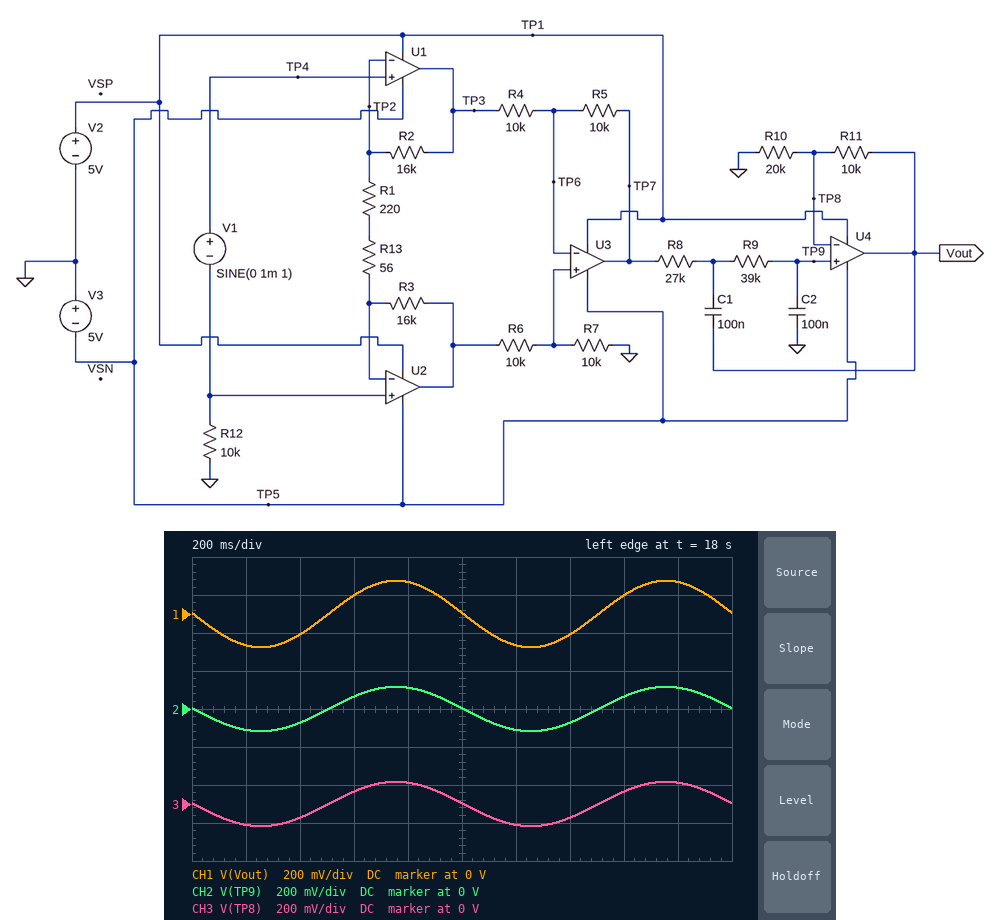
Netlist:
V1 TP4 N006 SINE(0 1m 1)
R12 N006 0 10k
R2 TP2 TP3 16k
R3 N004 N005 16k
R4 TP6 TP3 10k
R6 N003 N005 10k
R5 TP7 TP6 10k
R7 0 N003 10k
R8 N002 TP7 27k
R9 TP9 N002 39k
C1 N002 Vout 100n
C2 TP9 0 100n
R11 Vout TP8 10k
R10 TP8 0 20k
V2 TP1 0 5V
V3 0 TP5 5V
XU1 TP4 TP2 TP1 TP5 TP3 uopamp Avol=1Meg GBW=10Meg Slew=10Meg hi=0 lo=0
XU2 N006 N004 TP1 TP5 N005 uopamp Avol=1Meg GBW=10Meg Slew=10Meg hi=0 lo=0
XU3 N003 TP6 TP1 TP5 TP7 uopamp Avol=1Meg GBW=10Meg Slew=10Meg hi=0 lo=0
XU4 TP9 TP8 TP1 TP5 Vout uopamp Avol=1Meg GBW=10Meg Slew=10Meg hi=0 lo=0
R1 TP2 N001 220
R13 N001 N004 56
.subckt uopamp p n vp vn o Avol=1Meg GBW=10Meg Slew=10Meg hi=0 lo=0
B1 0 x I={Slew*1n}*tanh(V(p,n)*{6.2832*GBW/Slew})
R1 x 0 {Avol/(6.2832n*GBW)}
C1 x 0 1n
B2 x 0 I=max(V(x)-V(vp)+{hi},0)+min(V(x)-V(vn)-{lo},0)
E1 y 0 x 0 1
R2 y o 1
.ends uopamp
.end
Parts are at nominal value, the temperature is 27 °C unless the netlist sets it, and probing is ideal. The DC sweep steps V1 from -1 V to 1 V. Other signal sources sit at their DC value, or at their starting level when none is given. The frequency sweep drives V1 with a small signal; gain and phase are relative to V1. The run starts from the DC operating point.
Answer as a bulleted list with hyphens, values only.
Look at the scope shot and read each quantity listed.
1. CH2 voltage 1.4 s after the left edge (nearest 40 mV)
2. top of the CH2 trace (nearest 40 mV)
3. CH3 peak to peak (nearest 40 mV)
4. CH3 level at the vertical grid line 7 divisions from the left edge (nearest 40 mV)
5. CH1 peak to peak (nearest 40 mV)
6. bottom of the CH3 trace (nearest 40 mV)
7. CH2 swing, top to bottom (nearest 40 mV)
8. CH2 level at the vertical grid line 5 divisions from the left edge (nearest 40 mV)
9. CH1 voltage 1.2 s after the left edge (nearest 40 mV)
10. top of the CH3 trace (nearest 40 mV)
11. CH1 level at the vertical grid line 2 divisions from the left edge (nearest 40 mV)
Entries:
- -80 mV
- 120 mV
- 240 mV
- -80 mV
- 360 mV
- -120 mV
- 240 mV
- 0 V
- -160 mV
- 120 mV
- -120 mV
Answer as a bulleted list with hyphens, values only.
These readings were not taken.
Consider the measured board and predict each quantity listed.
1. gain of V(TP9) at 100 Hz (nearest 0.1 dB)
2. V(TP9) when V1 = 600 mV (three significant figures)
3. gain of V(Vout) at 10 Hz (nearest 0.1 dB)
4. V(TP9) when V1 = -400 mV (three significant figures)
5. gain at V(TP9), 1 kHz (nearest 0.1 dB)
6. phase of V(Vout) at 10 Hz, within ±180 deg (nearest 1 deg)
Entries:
- 28.2 dB
- -5.01 V
- 44.8 dB
- 5.01 V
- -11.0 dB
- 161 deg
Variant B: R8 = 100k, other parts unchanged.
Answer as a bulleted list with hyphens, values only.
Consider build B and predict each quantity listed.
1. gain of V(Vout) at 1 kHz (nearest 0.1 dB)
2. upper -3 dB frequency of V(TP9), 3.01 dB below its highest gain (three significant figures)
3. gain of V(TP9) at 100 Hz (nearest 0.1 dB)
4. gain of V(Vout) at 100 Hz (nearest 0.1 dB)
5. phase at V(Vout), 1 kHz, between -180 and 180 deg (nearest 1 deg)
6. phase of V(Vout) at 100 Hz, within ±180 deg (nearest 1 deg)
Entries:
- -18.9 dB
- 25.3 Hz
- 17.6 dB
- 21.1 dB
- 1 deg
- 21 deg
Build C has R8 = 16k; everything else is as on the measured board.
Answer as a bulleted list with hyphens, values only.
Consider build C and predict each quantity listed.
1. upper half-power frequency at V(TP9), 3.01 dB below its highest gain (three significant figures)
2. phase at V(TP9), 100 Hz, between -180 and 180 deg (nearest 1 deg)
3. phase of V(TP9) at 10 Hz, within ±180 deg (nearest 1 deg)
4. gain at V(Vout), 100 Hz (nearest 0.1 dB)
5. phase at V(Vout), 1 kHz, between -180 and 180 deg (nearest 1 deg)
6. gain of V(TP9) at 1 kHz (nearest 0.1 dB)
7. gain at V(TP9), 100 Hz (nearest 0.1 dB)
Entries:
- 44.7 Hz
- 64 deg
- 163 deg
- 34.5 dB
- 6 deg
- -6.5 dB
- 31.0 dB
